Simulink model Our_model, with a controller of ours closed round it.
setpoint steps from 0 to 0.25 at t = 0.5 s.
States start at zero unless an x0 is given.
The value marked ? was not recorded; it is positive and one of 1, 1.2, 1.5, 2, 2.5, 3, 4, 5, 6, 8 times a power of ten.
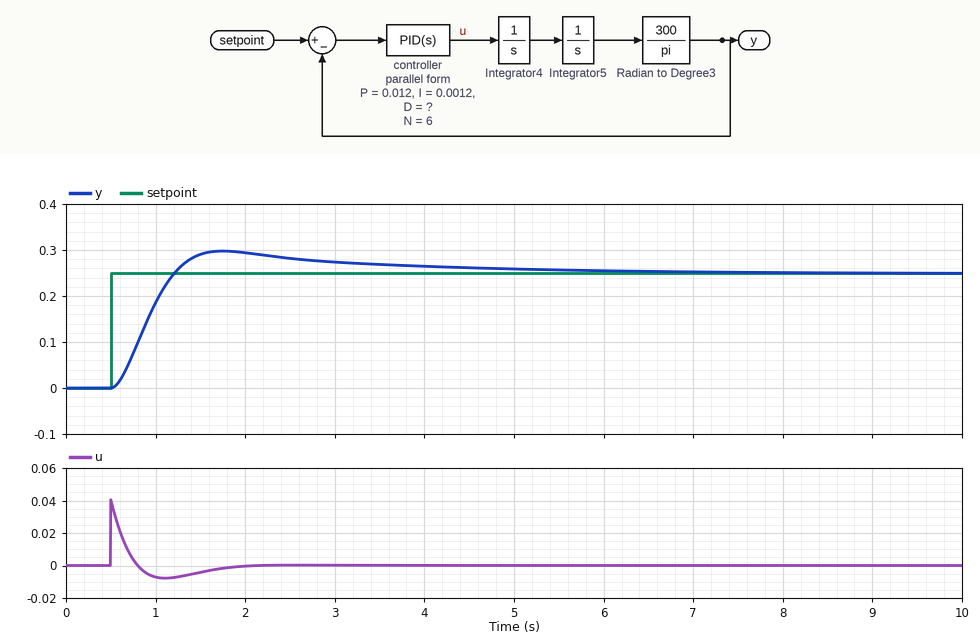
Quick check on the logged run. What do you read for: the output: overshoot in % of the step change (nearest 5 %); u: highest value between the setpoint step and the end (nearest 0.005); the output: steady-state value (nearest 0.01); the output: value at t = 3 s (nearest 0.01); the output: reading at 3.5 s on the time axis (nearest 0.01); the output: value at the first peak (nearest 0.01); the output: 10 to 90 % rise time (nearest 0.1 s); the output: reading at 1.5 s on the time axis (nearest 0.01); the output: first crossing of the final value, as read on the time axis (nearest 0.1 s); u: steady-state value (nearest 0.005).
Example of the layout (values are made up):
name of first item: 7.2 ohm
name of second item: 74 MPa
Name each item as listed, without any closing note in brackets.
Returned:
the output: overshoot in % of the step change: 20 %
u: highest value between the setpoint step and the end: 0.040
the output: steady-state value: 0.25
the output: value at t = 3 s: 0.27
the output: reading at 3.5 s on the time axis: 0.27
the output: value at the first peak: 0.30
the output: 10 to 90 % rise time: 0.5 s
the output: reading at 1.5 s on the time axis: 0.29
the output: first crossing of the final value, as read on the time axis: 1.2 s
u: steady-state value: 0.000
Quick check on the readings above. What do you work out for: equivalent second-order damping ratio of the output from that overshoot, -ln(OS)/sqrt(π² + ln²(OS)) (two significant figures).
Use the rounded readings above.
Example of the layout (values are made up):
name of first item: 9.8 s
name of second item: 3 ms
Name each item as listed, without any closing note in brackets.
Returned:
equivalent second-order damping ratio of the output from that overshoot, -ln(OS)/sqrt(π² + ln²(OS)): 0.46
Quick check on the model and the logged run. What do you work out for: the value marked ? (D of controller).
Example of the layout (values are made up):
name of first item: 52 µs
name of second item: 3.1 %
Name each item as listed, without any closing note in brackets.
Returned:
the value marked ?: 0.025
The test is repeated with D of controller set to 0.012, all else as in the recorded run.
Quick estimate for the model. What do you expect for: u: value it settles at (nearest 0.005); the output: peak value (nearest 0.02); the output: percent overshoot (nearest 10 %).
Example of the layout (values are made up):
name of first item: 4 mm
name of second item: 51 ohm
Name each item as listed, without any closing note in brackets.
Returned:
u: value it settles at: 0.000
the output: peak value: 0.34
the output: percent overshoot: 40 %
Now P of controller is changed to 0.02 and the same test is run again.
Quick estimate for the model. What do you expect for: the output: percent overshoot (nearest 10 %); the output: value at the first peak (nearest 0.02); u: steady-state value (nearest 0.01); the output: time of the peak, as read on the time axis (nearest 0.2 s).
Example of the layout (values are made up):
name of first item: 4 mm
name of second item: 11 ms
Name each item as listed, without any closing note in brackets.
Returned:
the output: percent overshoot: 30 %
the output: value at the first peak: 0.32
u: steady-state value: 0.00
the output: time of the peak, as read on the time axis: 1.6 s
